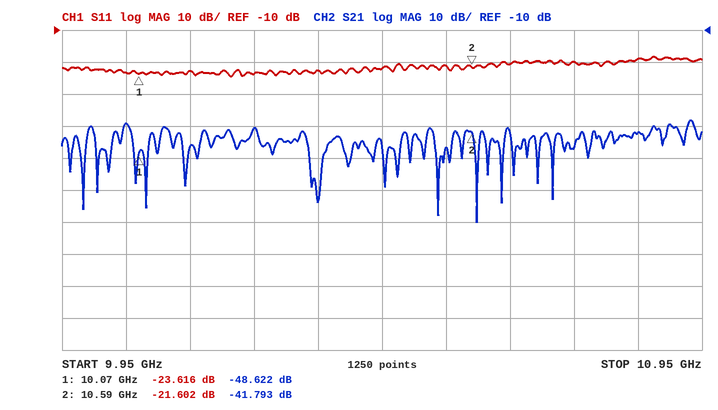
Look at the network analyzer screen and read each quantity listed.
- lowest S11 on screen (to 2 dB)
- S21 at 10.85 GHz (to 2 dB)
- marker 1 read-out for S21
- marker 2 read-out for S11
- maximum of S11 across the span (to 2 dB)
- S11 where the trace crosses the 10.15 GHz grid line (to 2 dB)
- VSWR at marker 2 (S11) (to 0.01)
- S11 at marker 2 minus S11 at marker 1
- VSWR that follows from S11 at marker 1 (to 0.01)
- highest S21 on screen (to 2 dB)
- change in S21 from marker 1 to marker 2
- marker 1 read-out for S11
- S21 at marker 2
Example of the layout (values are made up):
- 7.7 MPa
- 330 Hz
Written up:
- -24 dB
- -42 dB
- -48.622 dB
- -21.602 dB
- -18 dB
- -22 dB
- 1.18
- 2.014 dB
- 1.14
- -38 dB
- 6.829 dB
- -23.616 dB
- -41.793 dB
